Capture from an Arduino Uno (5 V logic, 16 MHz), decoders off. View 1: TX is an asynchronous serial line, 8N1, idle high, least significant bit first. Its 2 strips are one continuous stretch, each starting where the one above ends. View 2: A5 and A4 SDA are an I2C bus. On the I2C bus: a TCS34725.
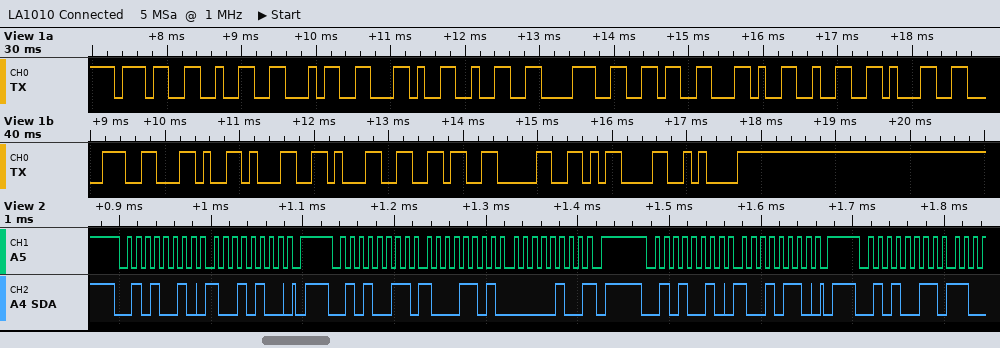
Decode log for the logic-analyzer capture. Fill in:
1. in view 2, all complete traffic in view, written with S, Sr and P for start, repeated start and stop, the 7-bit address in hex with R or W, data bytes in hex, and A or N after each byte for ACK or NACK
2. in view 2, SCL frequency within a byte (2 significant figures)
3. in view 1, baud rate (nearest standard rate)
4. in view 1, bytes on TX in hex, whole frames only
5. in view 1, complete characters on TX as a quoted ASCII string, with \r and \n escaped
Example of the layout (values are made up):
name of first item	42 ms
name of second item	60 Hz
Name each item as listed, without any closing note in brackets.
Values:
in view 2, all complete traffic in view, written with S, Sr and P for start, repeated start and stop, the 7-bit address in hex with R or W, data bytes in hex, and A or N after each byte for ACK or NACK	S 29W A 94 A P S 29R A 8D A 04 N P S 29W A 96 A P S 29R A
in view 2, SCL frequency within a byte	100 kHz
in view 1, baud rate	9600 baud
in view 1, bytes on TX in hex, whole frames only	37 32 34 2C 32 38 36 2C 32 31 38 2C 31 31 36 30 0D 0A
in view 1, complete characters on TX as a quoted ASCII string, with \r and \n escaped	"724,286,218,1160\r\n"
